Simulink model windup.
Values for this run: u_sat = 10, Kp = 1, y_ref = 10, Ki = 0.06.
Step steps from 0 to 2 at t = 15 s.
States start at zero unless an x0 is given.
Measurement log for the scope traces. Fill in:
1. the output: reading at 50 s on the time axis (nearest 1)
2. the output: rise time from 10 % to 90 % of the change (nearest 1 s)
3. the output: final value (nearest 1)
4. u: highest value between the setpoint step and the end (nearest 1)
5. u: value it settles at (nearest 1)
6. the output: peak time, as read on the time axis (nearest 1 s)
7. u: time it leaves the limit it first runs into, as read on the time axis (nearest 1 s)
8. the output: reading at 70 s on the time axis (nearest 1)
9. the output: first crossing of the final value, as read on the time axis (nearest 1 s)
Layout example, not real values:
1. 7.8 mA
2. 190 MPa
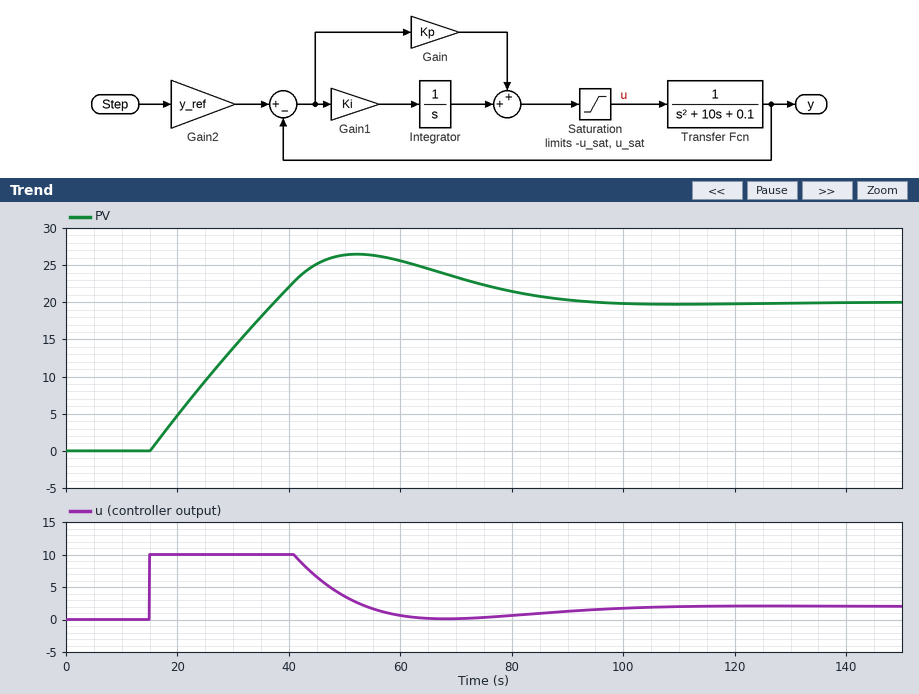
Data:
1. 26
2. 18 s
3. 20
4. 10
5. 2
6. 52 s
7. 41 s
8. 23
9. 37 s
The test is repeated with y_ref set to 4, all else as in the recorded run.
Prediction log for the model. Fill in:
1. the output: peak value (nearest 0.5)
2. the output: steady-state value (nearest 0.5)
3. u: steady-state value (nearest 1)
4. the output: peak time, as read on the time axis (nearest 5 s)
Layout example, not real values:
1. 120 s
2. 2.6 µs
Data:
1. 9.5
2. 8.0
3. 1
4. 45 s
